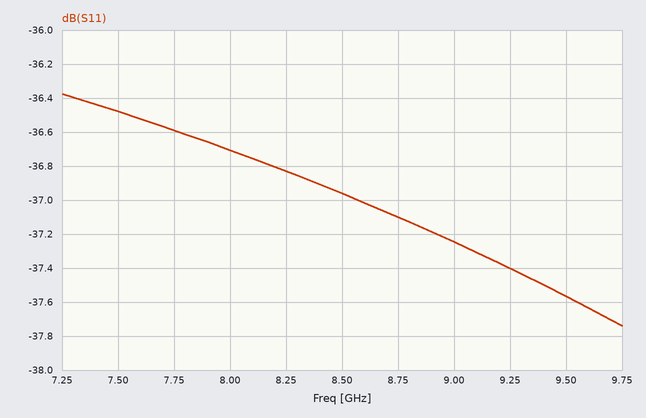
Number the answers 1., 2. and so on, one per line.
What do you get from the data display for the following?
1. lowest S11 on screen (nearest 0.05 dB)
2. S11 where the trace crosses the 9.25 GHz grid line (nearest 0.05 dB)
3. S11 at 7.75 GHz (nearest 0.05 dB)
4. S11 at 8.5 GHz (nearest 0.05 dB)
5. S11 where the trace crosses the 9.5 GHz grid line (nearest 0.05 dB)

1. -37.75 dB
2. -37.40 dB
3. -36.60 dB
4. -36.95 dB
5. -37.55 dB
